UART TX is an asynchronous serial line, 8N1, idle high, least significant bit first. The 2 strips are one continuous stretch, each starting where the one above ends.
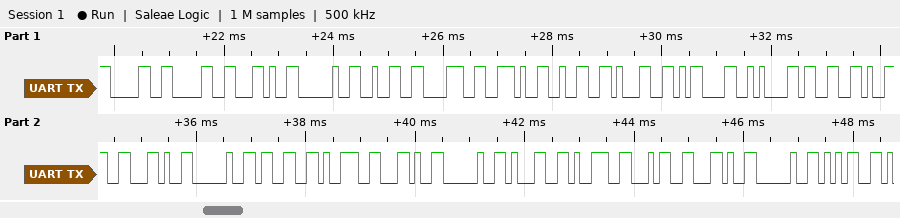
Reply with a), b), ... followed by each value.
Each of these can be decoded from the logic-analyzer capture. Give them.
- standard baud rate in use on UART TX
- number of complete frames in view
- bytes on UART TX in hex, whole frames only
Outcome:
a) 9600 baud
b) 25
c) 30 30 2C 20 32 38 2E 32 31 0D 0A 33 39 2C 20 33 39 2C 20 31 39 34 2C 20 35
